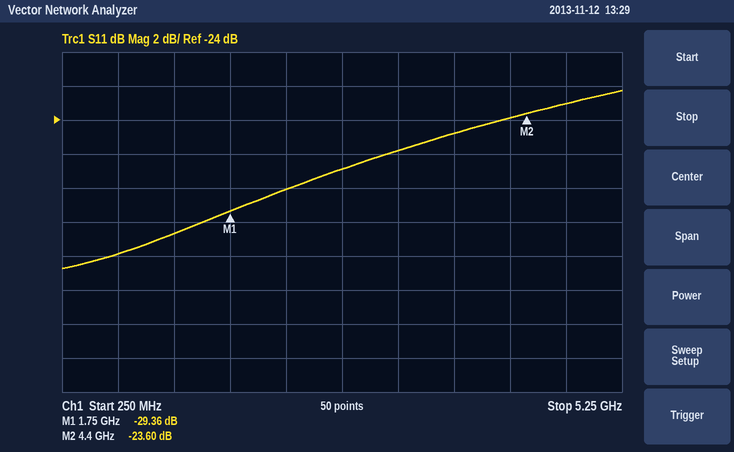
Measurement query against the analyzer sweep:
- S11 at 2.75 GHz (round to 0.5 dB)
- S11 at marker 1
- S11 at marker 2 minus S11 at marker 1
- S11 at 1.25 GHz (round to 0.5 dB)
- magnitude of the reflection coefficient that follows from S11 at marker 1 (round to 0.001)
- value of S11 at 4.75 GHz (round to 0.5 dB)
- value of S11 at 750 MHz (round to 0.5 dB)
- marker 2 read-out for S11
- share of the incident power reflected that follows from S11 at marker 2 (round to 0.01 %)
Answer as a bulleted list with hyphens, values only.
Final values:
- -27.0 dB
- -29.36 dB
- 5.76 dB
- -30.5 dB
- 0.034
- -23.0 dB
- -32.0 dB
- -23.60 dB
- 0.44 %
